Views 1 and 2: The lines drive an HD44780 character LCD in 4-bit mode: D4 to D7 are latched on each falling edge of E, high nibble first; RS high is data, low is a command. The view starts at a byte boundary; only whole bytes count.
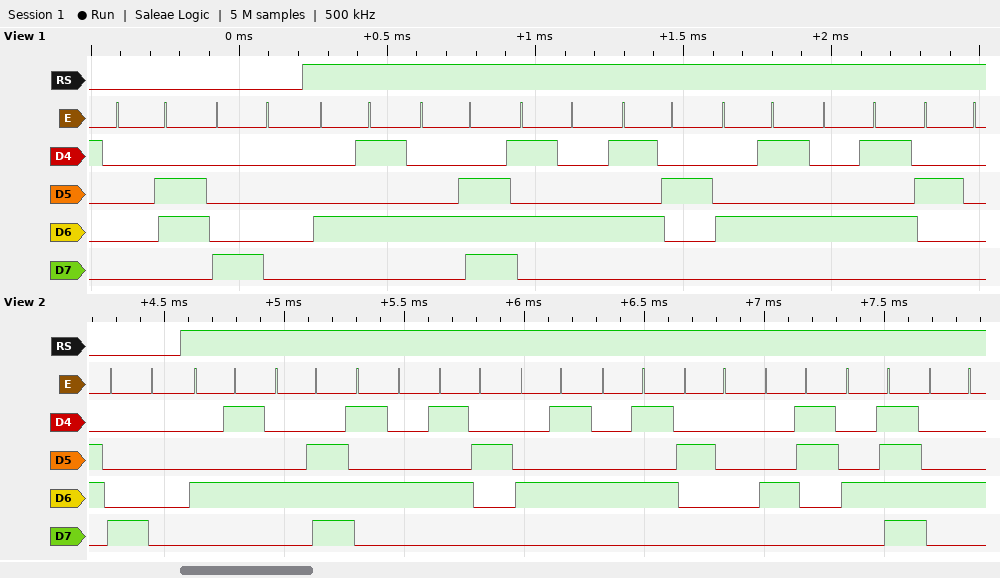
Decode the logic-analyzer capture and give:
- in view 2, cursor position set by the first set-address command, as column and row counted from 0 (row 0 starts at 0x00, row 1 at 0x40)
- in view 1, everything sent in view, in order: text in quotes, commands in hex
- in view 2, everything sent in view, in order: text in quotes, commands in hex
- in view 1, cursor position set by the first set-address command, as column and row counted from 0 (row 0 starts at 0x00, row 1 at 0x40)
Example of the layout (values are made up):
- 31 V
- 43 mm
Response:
- column 0, row 0
- 0x06 0x80 "ENTREE "
- 0x80 "ENTREE COD"
- column 0, row 0
